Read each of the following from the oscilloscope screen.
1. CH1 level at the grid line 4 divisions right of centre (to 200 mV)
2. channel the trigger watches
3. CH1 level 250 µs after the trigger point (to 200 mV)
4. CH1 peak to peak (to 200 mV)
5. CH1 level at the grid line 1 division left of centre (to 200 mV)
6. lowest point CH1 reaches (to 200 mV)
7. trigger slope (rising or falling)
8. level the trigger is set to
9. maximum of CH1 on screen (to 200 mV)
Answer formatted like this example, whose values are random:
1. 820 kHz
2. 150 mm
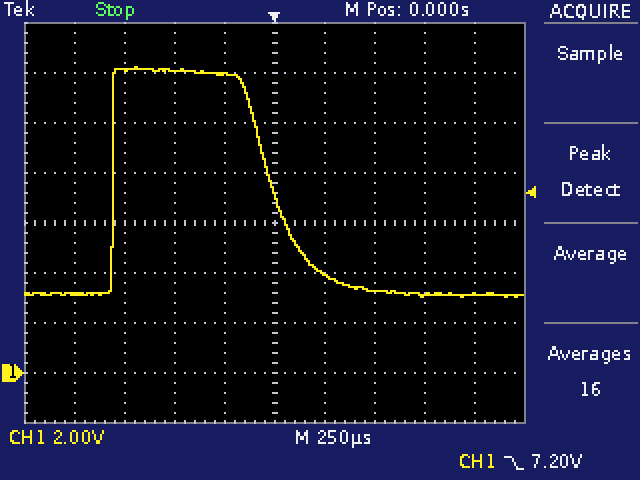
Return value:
1. 3.2 V
2. CH1
3. 4.0 V
4. 9.2 V
5. 12.0 V
6. 3.0 V
7. falling
8. 7.20 V
9. 12.2 V
